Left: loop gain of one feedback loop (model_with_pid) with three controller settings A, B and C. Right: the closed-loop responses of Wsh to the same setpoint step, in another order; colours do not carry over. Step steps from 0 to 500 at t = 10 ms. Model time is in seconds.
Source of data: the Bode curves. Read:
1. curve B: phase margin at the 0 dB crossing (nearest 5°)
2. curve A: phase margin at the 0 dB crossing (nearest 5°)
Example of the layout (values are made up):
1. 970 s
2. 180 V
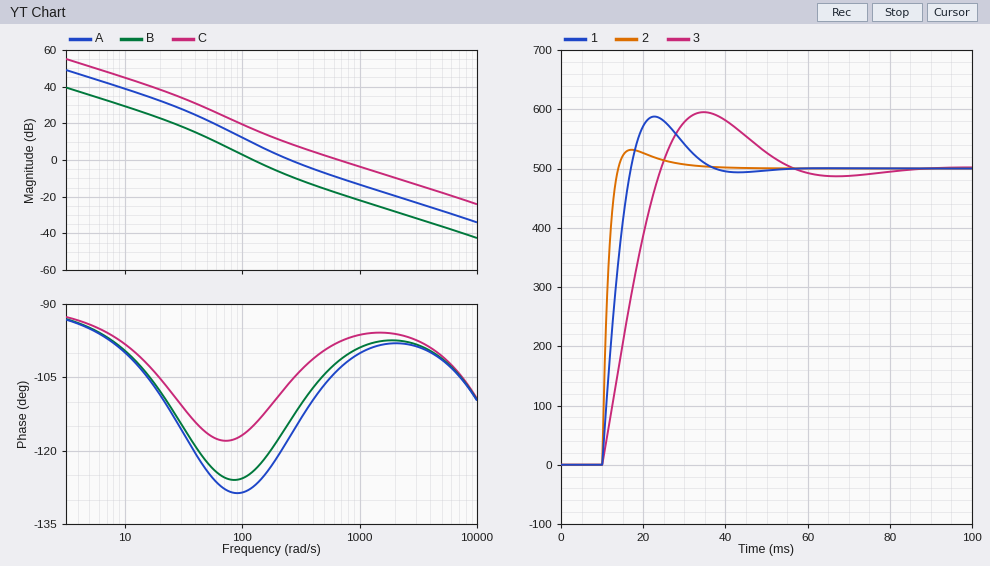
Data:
1. 55°
2. 65°
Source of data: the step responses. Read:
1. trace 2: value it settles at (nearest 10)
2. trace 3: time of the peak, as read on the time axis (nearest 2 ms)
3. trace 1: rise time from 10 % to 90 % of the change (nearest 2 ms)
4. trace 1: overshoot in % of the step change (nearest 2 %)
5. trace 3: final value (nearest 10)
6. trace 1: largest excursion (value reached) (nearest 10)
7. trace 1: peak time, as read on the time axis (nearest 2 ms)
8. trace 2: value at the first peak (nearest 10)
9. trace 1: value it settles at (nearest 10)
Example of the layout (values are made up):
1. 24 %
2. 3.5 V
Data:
1. 500
2. 34 ms
3. 6 ms
4. 18 %
5. 500
6. 590
7. 22 ms
8. 530
9. 500
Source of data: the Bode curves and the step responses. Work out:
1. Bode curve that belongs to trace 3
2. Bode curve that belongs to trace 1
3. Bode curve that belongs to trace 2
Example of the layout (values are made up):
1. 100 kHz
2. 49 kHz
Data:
1. B
2. A
3. C
